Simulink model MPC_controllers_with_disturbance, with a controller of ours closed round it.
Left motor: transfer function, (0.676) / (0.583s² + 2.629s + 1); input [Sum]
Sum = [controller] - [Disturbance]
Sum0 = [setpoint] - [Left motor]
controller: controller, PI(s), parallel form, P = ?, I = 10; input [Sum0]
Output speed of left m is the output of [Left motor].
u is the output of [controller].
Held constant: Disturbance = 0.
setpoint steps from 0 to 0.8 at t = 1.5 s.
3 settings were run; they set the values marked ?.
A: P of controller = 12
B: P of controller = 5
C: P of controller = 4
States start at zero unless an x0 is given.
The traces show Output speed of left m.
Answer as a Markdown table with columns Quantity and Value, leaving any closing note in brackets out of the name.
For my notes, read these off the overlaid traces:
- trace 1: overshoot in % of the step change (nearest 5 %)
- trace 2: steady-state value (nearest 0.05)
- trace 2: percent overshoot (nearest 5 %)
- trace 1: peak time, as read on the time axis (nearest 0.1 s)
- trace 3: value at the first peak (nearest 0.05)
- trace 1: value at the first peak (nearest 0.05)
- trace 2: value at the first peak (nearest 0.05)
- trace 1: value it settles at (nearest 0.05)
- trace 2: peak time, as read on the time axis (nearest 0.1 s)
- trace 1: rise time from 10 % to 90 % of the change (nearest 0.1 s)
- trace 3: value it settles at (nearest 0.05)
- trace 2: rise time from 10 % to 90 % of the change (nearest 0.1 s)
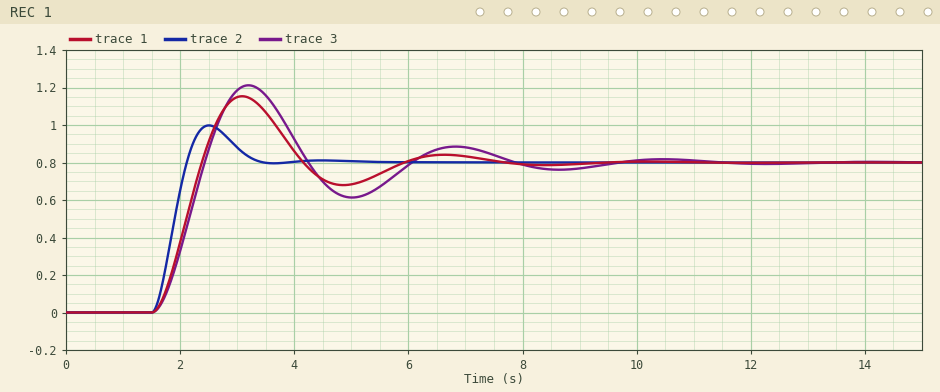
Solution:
| Quantity | Value |
|---|---|
| trace 1: overshoot in % of the step change | 45 % |
| trace 2: steady-state value | 0.80 |
| trace 2: percent overshoot | 25 % |
| trace 1: peak time, as read on the time axis | 3.1 s |
| trace 3: value at the first peak | 1.20 |
| trace 1: value at the first peak | 1.15 |
| trace 2: value at the first peak | 1.00 |
| trace 1: value it settles at | 0.80 |
| trace 2: peak time, as read on the time axis | 2.5 s |
| trace 1: rise time from 10 % to 90 % of the change | 0.6 s |
| trace 3: value it settles at | 0.80 |
| trace 2: rise time from 10 % to 90 % of the change | 0.4 s |
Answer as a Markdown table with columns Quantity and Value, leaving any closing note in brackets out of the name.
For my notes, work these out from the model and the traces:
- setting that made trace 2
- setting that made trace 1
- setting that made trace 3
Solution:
| Quantity | Value |
|---|---|
| setting that made trace 2 | A |
| setting that made trace 1 | B |
| setting that made trace 3 | C |
